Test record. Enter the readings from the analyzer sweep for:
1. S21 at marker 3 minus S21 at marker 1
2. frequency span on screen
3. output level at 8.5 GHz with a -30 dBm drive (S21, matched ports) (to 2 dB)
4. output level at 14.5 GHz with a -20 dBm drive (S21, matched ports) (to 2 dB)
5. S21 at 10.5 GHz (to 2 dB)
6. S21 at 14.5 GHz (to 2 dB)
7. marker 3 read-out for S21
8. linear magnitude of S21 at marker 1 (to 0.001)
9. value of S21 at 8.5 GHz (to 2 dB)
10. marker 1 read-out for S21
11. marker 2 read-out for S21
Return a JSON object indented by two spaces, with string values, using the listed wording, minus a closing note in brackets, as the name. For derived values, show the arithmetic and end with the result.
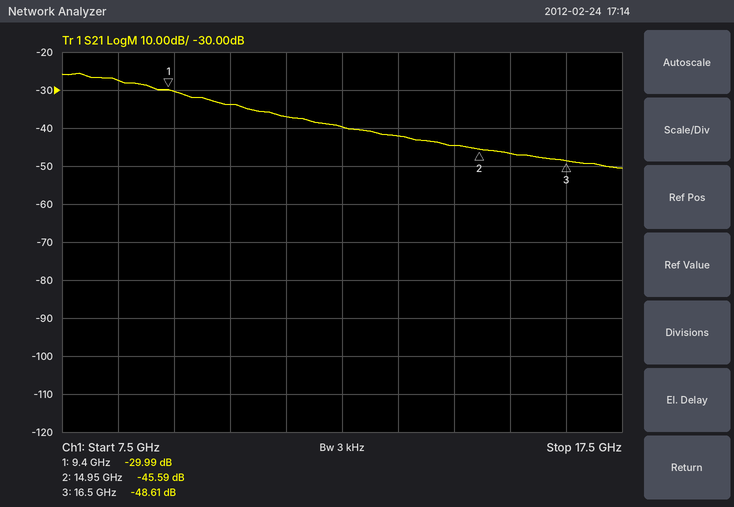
{
  "S21 at marker 3 minus S21 at marker 1": "-48.61 − (-29.99) = -18.62 dB",
  "frequency span on screen": "10 GHz",
  "output level at 8.5 GHz with a -30 dBm drive (S21, matched ports)": "-30 dBm + (-28 dB) = -58 dBm",
  "output level at 14.5 GHz with a -20 dBm drive (S21, matched ports)": "-20 dBm + (-44 dB) = -64 dBm",
  "S21 at 10.5 GHz": "-34 dB",
  "S21 at 14.5 GHz": "-44 dB",
  "marker 3 read-out for S21": "-48.61 dB",
  "linear magnitude of S21 at marker 1": "10^(-29.99/20) ≈ 0.032",
  "value of S21 at 8.5 GHz": "-28 dB",
  "marker 1 read-out for S21": "-29.99 dB",
  "marker 2 read-out for S21": "-45.59 dB"
}
